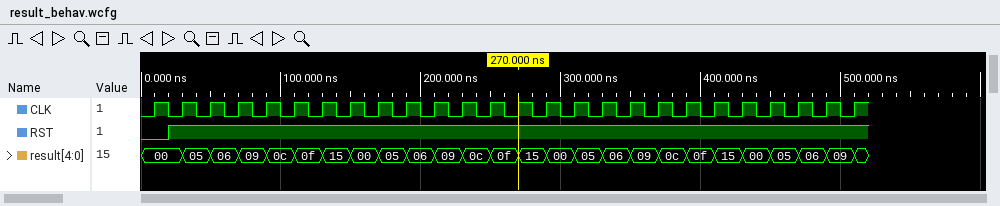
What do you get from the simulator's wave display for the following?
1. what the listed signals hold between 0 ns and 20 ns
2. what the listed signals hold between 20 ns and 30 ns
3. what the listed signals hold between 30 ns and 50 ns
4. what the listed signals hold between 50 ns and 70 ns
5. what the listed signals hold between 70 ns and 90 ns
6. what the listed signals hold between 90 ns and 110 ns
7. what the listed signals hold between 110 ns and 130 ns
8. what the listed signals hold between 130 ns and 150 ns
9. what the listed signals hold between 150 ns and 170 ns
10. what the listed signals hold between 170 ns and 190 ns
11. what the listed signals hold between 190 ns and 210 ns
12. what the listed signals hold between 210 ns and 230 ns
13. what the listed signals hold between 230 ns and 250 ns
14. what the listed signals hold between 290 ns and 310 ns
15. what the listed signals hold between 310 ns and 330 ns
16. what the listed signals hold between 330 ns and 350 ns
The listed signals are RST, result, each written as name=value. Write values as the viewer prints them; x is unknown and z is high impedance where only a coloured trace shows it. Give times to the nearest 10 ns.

RST=0, result=00
RST=1, result=00
RST=1, result=05
RST=1, result=06
RST=1, result=09
RST=1, result=0c
RST=1, result=0f
RST=1, result=15
RST=1, result=00
RST=1, result=05
RST=1, result=06
RST=1, result=09
RST=1, result=0c
RST=1, result=00
RST=1, result=05
RST=1, result=06
